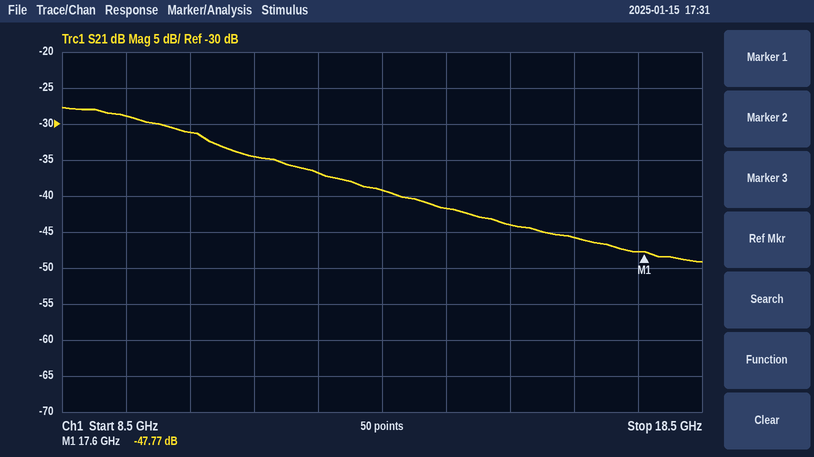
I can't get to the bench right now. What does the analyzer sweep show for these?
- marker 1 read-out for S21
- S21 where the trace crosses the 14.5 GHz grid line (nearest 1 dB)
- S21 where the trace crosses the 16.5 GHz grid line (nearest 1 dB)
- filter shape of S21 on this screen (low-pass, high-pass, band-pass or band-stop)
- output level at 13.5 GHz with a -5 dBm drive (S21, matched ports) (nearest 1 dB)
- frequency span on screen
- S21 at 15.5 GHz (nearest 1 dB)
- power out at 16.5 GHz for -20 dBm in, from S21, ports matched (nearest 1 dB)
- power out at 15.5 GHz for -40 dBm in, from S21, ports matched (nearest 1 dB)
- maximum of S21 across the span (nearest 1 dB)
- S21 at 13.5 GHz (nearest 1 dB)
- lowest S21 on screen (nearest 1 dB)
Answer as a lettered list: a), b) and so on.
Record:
a) -47.77 dB
b) -42 dB
c) -46 dB
d) low-pass
e) -44 dBm
f) 10 GHz
g) -44 dB
h) -66 dBm
i) -84 dBm
j) -28 dB
k) -39 dB
l) -49 dB
